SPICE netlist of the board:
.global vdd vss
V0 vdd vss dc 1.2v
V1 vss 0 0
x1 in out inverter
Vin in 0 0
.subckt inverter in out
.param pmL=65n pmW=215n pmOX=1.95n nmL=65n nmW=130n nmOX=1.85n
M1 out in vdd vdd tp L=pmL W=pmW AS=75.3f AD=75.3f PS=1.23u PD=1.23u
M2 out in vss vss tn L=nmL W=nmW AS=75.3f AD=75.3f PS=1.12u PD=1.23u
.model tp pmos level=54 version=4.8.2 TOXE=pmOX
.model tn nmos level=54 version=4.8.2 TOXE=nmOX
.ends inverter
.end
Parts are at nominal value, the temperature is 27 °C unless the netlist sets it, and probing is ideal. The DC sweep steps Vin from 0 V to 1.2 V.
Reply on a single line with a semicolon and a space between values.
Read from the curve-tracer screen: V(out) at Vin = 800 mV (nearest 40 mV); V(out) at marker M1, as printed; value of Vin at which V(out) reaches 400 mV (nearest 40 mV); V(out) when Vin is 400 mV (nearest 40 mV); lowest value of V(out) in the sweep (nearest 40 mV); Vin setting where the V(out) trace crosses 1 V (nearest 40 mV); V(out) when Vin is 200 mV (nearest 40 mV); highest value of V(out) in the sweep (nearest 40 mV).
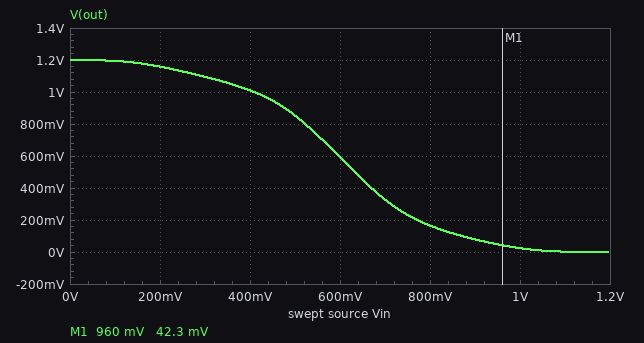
160 mV; 42.3 mV; 680 mV; 1.00 V; 0 V; 400 mV; 1.16 V; 1.20 V
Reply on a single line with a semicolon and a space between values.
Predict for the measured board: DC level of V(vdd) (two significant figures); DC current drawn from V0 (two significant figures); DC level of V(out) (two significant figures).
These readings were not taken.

1.2 V; 130 nA; 1.2 V
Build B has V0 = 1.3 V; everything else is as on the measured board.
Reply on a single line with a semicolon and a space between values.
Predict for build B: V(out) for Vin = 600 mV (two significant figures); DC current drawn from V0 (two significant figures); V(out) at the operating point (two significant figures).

790 mV; 150 nA; 1.3 V
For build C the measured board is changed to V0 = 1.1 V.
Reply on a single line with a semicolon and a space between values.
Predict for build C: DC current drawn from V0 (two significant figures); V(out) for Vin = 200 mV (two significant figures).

110 nA; 1.1 V
